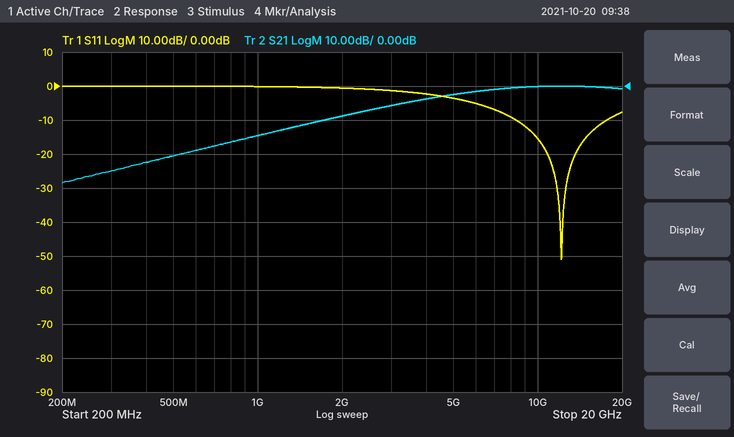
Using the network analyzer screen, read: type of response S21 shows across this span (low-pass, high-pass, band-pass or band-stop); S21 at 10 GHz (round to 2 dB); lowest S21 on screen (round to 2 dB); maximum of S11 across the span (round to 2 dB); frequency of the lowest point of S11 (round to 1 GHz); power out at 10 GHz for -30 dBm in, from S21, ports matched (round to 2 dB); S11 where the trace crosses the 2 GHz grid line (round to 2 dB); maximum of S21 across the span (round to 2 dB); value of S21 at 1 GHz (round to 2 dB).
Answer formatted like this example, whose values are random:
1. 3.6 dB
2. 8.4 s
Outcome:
1. high-pass
2. 0 dB
3. -28 dB
4. 0 dB
5. 12 GHz
6. -30 dBm
7. 0 dB
8. 0 dB
9. -14 dB
